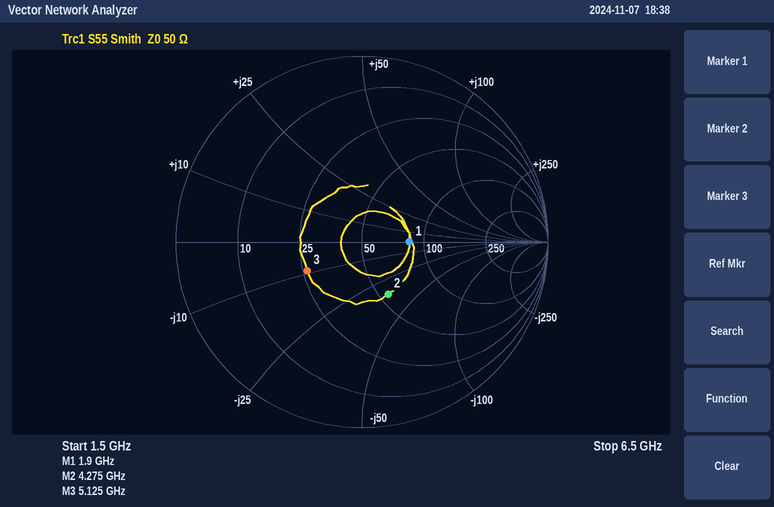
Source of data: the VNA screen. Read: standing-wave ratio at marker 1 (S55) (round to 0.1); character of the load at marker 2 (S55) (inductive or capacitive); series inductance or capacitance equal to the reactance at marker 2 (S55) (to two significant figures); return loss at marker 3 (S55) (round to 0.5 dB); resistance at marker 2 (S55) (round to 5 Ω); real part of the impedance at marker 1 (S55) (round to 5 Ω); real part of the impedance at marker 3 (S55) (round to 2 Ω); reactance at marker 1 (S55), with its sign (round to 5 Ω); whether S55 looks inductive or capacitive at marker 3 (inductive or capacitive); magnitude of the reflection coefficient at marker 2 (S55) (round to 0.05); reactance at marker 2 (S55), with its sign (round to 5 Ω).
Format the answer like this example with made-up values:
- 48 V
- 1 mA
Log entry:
- 1.7
- capacitive
- 1.1 pF
- 9.5 dB
- 55 Ω
- 85 Ω
- 26 Ω
- 0 Ω
- capacitive
- 0.30
- -35 Ω
